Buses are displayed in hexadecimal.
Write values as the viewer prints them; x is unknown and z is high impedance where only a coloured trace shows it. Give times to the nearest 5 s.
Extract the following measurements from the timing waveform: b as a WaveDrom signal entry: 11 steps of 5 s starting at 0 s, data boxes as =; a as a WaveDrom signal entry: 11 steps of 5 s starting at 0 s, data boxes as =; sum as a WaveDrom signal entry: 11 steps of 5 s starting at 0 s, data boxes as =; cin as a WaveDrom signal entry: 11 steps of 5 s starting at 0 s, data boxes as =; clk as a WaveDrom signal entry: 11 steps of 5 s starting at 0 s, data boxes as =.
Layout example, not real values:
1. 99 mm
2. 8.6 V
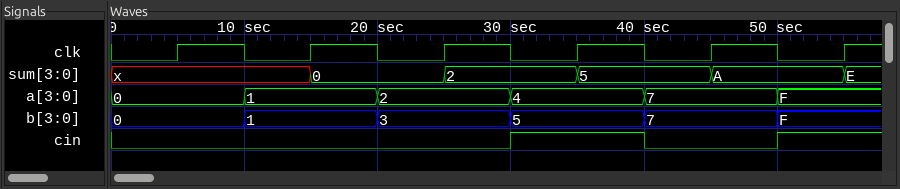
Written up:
1. {name: 'b', wave: '=.=.=.=.=.=', data: '0 1 3 5 7 F'}
2. {name: 'a', wave: '=.=.=.=.=.=', data: '0 1 2 4 7 F'}
3. {name: 'sum', wave: 'x..=.=.=.=.', data: '0 2 5 A'}
4. {name: 'cin', wave: '0.....1.0.1'}
5. {name: 'clk', wave: '01010101010'}
